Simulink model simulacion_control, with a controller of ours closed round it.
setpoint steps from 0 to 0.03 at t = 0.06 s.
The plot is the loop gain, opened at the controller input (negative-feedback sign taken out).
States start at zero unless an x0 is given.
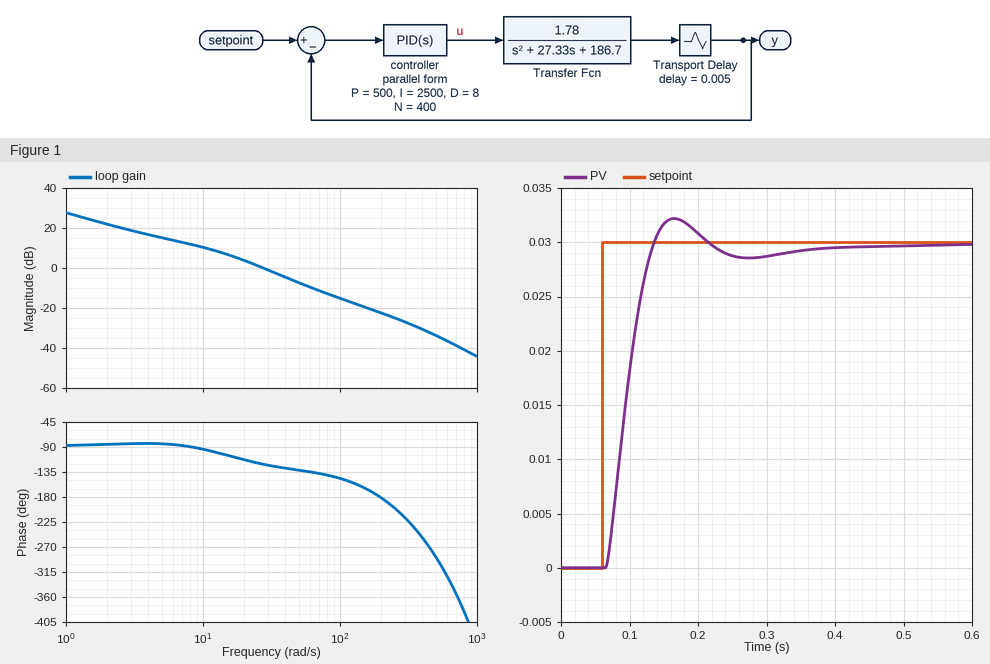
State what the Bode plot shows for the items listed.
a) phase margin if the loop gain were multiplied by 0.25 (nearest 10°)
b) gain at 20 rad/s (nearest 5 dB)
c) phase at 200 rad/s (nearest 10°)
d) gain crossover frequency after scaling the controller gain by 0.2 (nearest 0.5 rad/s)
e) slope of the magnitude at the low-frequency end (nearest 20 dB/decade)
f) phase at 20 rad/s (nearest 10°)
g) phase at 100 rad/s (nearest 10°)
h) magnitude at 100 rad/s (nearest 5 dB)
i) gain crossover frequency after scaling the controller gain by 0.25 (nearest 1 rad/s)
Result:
90°
5 dB
-180°
6.0 rad/s
-20 dB/decade
-110°
-150°
-15 dB
8 rad/s
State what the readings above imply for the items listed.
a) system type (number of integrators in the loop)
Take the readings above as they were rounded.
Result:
1
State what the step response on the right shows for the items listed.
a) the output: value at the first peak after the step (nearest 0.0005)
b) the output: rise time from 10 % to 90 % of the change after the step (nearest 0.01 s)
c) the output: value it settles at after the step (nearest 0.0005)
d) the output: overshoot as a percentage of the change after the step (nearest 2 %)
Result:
0.0320
0.05 s
0.0300
8 %
